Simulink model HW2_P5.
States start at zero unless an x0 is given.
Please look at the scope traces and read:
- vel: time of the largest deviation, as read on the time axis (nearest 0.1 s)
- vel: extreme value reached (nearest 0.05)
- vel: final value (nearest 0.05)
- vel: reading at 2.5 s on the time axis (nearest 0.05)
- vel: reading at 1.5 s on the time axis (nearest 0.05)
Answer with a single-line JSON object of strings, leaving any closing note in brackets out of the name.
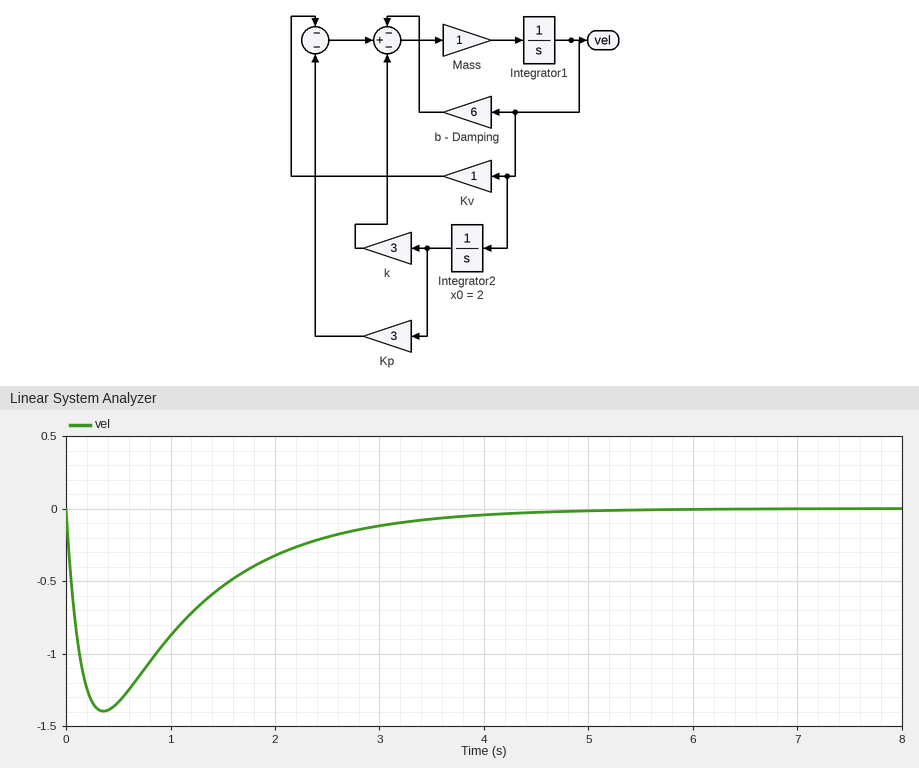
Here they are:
{"vel: time of the largest deviation, as read on the time axis": "0.4 s", "vel: extreme value reached": "-1.40", "vel: final value": "0.00", "vel: reading at 2.5 s on the time axis": "-0.20", "vel: reading at 1.5 s on the time axis": "-0.55"}
